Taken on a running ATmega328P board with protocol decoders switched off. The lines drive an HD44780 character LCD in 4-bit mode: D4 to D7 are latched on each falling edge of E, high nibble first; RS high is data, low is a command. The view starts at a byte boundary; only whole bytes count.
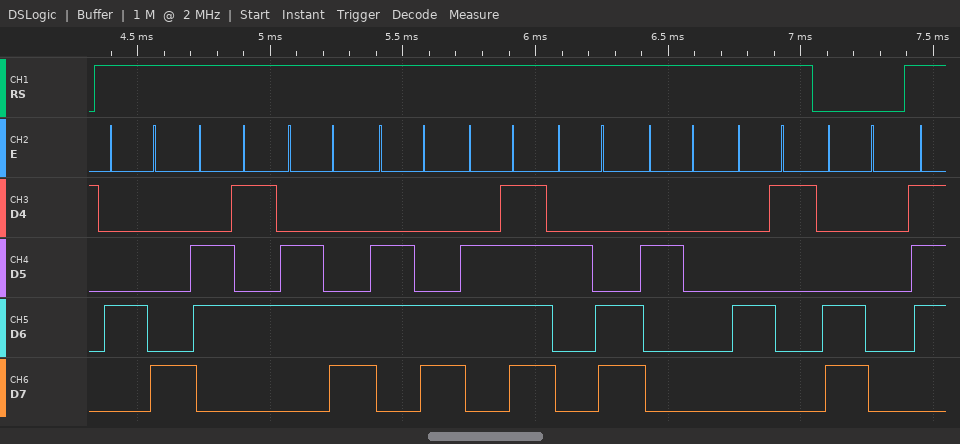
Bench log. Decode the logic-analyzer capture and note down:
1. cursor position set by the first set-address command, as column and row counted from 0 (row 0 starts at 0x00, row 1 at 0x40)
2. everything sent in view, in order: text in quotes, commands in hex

column 0, row 1
"Hello, A" 0xC0
